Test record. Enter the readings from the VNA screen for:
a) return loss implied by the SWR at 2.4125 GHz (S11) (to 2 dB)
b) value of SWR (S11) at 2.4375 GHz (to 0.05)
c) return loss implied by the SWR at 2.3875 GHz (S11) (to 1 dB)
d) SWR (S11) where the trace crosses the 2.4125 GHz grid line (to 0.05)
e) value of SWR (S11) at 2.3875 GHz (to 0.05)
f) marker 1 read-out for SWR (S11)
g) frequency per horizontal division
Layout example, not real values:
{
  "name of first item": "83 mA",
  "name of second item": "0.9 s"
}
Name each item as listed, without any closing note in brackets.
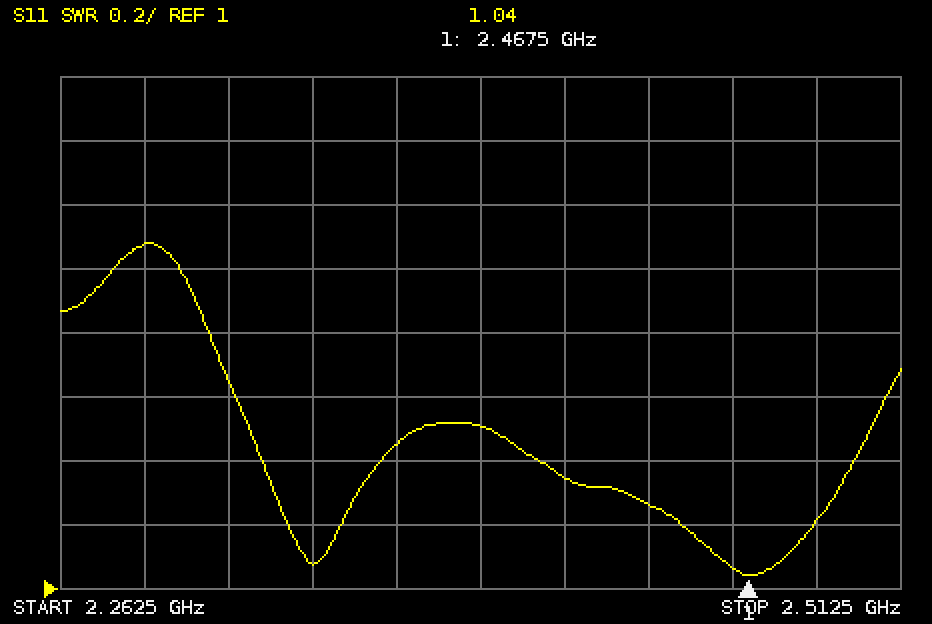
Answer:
{
  "return loss implied by the SWR at 2.4125 GHz (S11)": "16 dB",
  "value of SWR (S11) at 2.4375 GHz": "1.25",
  "return loss implied by the SWR at 2.3875 GHz (S11)": "14 dB",
  "SWR (S11) where the trace crosses the 2.4125 GHz grid line": "1.35",
  "value of SWR (S11) at 2.3875 GHz": "1.50",
  "marker 1 read-out for SWR": "1.04",
  "frequency per horizontal division": "25 MHz"
}
